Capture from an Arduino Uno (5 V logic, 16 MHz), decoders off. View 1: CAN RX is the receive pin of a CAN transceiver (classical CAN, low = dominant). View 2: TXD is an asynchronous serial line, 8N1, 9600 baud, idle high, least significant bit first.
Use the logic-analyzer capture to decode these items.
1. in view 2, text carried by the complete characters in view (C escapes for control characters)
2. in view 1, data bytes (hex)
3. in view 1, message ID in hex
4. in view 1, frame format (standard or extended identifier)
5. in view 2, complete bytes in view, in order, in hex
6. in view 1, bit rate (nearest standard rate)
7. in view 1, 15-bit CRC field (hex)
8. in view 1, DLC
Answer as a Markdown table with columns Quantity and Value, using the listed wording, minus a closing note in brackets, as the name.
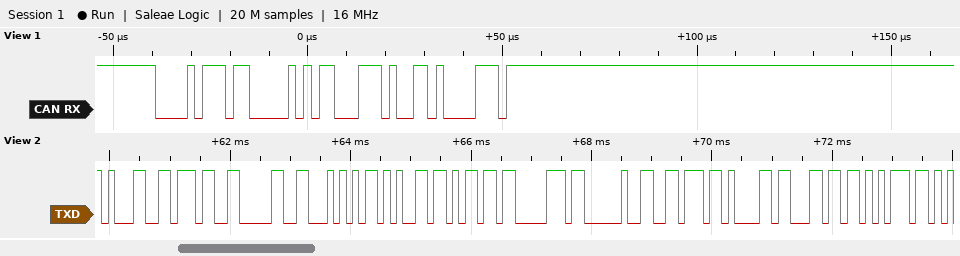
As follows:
| Quantity | Value |
|---|---|
| in view 2, text carried by the complete characters in view | "170Temp valu" |
| in view 1, data bytes | 63 |
| in view 1, message ID in hex | 0x0BB |
| in view 1, frame format | standard |
| in view 2, complete bytes in view, in order, in hex | 0x31 0x37 0x30 0x54 0x65 0x6D 0x70 0x20 0x76 0x61 0x6C 0x75 |
| in view 1, bit rate | 500 kbit/s |
| in view 1, 15-bit CRC field | 0x5343 |
| in view 1, DLC | 1 |
